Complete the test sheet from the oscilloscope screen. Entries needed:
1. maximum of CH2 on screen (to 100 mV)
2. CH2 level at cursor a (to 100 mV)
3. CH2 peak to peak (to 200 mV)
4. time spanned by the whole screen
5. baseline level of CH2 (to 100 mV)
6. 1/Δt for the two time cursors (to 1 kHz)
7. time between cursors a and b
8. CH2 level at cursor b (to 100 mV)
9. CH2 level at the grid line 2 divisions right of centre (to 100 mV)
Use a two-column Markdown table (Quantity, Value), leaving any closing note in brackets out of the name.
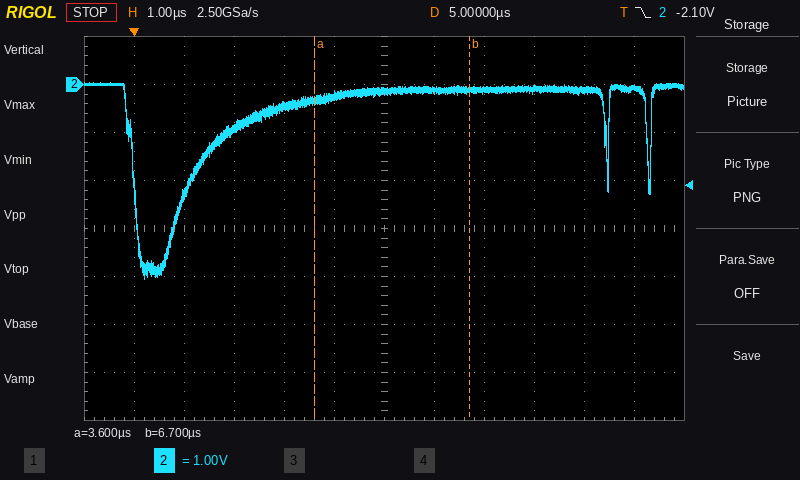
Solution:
| Quantity | Value |
|---|---|
| maximum of CH2 on screen | 0.0 V |
| CH2 level at cursor a | -300 mV |
| CH2 peak to peak | 4.0 V |
| time spanned by the whole screen | 12 µs |
| baseline level of CH2 | -100 mV |
| 1/Δt for the two time cursors | 323 kHz |
| time between cursors a and b | 3.1 µs |
| CH2 level at cursor b | -100 mV |
| CH2 level at the grid line 2 divisions right of centre | -100 mV |
